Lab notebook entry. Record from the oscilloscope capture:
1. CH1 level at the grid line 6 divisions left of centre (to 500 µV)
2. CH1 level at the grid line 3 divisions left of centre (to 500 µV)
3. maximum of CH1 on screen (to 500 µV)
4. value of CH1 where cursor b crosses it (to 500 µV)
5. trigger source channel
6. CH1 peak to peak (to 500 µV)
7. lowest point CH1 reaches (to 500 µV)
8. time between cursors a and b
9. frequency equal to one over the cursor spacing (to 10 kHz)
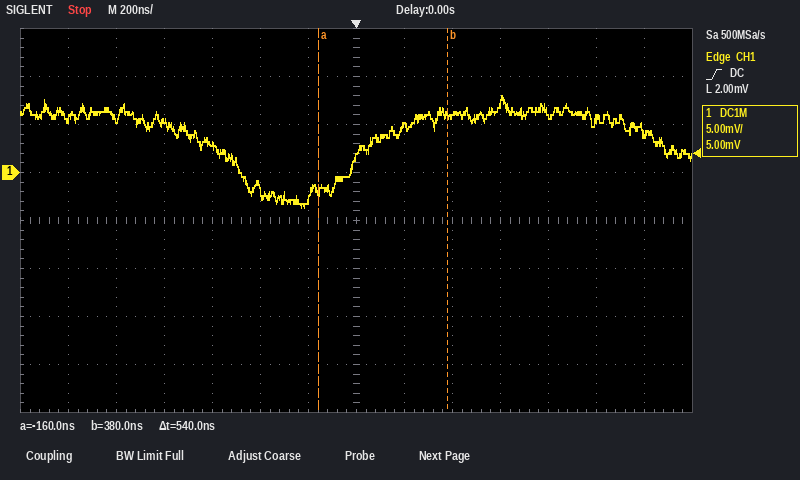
5.5 mV
3.0 mV
8.0 mV
6.0 mV
CH1
11.5 mV
-3.5 mV
540 ns
1.85 MHz
